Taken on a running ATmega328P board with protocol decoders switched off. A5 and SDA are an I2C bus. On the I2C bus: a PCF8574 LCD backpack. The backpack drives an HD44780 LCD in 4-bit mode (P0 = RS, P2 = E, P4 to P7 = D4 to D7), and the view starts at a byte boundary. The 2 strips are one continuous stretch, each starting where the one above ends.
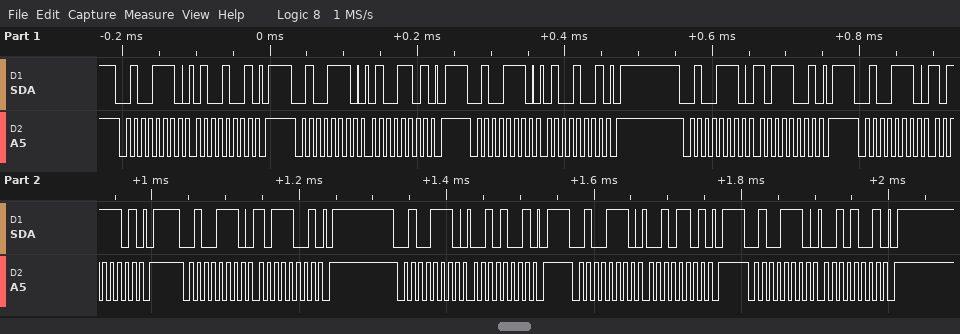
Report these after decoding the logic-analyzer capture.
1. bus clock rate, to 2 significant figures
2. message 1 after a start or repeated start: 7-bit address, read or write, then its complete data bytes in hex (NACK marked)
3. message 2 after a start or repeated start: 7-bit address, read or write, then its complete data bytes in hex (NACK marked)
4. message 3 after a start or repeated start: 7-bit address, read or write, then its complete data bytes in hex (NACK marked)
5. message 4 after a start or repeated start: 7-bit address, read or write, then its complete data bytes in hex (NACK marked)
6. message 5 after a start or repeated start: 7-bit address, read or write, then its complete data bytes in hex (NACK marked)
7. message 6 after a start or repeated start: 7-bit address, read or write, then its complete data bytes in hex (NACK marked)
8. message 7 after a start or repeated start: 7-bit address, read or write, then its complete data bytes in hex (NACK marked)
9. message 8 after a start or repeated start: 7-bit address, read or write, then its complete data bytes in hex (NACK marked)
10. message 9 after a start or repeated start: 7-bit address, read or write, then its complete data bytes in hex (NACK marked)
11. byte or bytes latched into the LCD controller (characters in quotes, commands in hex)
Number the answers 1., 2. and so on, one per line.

1. 100 kHz
2. 0x27 write: 49
3. 0x27 write: 4D
4. 0x27 write: 49
5. 0x27 write: B9
6. 0x27 write: BD
7. 0x27 write: B9
8. 0x27 write: 29
9. 0x27 write: 2D
10. 0x27 write: 29
11. 'K'
